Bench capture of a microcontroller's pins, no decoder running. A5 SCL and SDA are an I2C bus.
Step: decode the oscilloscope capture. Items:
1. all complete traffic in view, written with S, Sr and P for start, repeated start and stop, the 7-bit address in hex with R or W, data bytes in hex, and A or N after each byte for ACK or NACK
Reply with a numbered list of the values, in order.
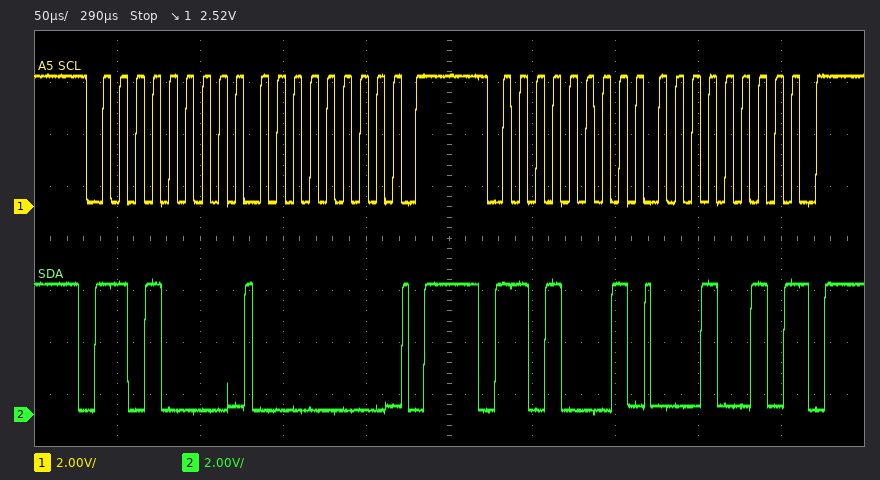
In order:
1. S 68W A 00 A P S 68R A 12 N P
